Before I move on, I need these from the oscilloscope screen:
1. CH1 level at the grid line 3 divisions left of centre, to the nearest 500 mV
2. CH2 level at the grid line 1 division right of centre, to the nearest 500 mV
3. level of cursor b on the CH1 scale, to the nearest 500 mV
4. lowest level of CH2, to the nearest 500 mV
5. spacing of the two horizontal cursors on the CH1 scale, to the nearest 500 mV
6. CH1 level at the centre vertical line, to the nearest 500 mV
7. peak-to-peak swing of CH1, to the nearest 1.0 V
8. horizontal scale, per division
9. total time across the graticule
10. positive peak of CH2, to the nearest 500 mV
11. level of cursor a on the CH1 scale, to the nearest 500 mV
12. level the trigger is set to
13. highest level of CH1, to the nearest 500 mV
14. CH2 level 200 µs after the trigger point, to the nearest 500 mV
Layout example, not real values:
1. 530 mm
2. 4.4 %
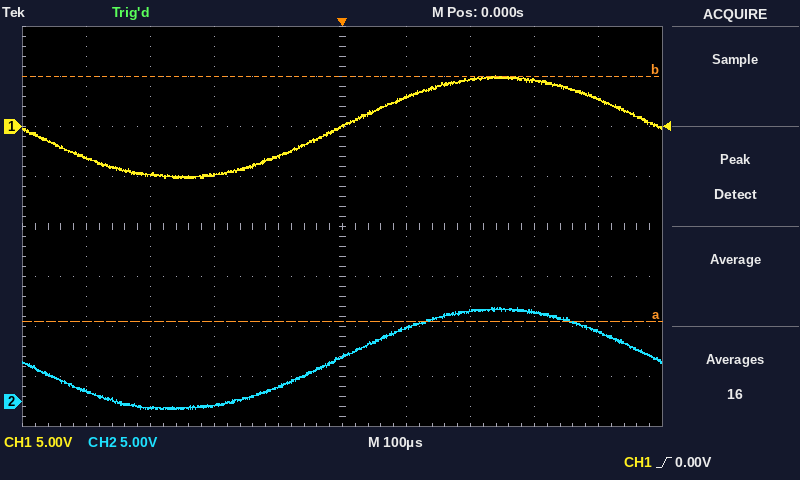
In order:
1. -5.0 V
2. 7.5 V
3. 5.0 V
4. -1.0 V
5. 24.5 V
6. 0.0 V
7. 10.0 V
8. 100 µs
9. 1 ms
10. 9.5 V
11. -19.5 V
12. 0.00 V
13. 5.0 V
14. 9.0 V
